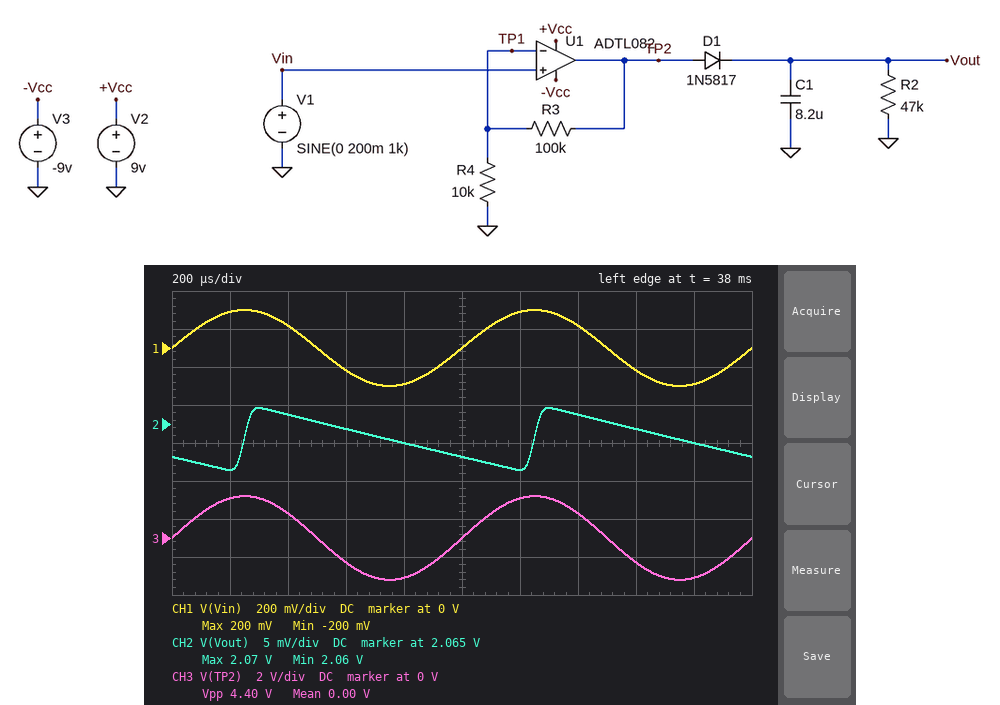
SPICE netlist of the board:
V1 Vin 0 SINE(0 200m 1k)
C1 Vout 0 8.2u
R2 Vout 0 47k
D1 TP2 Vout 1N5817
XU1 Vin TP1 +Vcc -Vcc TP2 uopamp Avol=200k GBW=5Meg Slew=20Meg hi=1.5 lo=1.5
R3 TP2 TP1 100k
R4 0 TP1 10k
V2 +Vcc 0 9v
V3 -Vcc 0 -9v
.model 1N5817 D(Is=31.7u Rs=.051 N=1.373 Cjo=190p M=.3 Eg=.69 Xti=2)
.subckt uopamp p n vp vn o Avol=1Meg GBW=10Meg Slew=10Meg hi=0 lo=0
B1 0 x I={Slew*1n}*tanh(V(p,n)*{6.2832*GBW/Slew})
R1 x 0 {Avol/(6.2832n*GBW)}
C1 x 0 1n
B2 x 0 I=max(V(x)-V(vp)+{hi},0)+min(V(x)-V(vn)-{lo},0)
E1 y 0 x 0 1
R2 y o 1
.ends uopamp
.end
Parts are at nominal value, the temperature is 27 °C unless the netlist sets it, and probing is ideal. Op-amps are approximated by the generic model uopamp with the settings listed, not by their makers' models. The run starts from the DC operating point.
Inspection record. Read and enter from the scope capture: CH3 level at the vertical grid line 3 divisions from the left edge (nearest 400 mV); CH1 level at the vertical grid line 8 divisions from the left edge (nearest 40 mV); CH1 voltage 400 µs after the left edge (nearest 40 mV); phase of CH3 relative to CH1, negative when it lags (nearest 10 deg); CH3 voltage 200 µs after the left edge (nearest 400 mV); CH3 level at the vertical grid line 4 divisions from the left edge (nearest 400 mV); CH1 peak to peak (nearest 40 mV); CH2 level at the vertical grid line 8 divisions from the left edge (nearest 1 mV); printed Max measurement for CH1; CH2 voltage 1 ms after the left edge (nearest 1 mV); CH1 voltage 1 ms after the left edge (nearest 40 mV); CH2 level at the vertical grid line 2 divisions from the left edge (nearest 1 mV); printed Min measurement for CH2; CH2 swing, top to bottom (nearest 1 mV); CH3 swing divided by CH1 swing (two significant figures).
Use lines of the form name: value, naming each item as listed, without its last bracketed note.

CH3 level at the vertical grid line 3 divisions from the left edge: -1.2 V
CH1 level at the vertical grid line 8 divisions from the left edge: -120 mV
CH1 voltage 400 µs after the left edge: 120 mV
phase of CH3 relative to CH1, negative when it lags: 0 deg
CH3 voltage 200 µs after the left edge: 2.0 V
CH3 level at the vertical grid line 4 divisions from the left edge: -2.0 V
CH1 peak to peak: 400 mV
CH2 level at the vertical grid line 8 divisions from the left edge: 2.064 V
printed Max measurement for CH1: 200 mV
CH2 voltage 1 ms after the left edge: 2.061 V
CH1 voltage 1 ms after the left edge: 0 V
CH2 level at the vertical grid line 2 divisions from the left edge: 2.066 V
printed Min measurement for CH2: 2.06 V
CH2 swing, top to bottom: 8 mV
CH3 swing divided by CH1 swing: 11
